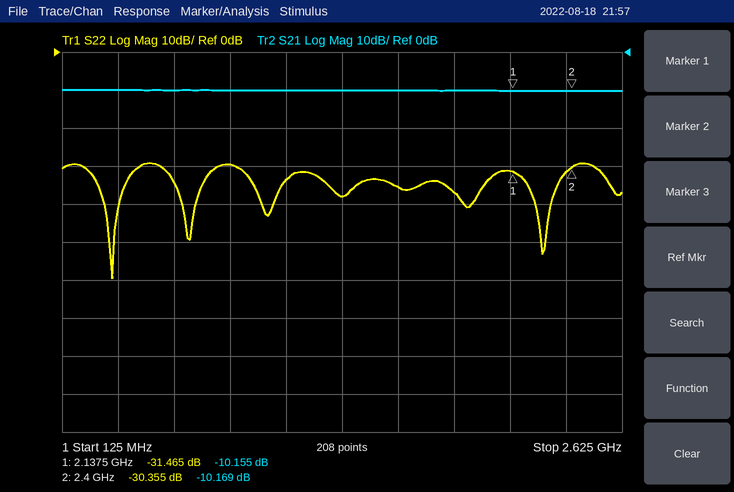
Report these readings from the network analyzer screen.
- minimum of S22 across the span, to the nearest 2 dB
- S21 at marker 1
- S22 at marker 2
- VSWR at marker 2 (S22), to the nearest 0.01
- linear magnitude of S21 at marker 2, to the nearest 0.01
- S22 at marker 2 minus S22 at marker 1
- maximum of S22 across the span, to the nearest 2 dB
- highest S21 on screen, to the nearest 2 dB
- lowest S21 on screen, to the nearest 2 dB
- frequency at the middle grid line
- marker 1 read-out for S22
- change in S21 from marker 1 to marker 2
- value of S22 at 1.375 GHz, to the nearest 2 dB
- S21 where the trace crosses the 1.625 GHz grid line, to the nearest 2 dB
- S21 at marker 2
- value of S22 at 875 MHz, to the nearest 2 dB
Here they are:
-60 dB
-10.155 dB
-30.355 dB
1.06
0.31
1.110 dB
-30 dB
-10 dB
-10 dB
1.375 GHz
-31.465 dB
-0.014 dB
-38 dB
-10 dB
-10.169 dB
-30 dB
